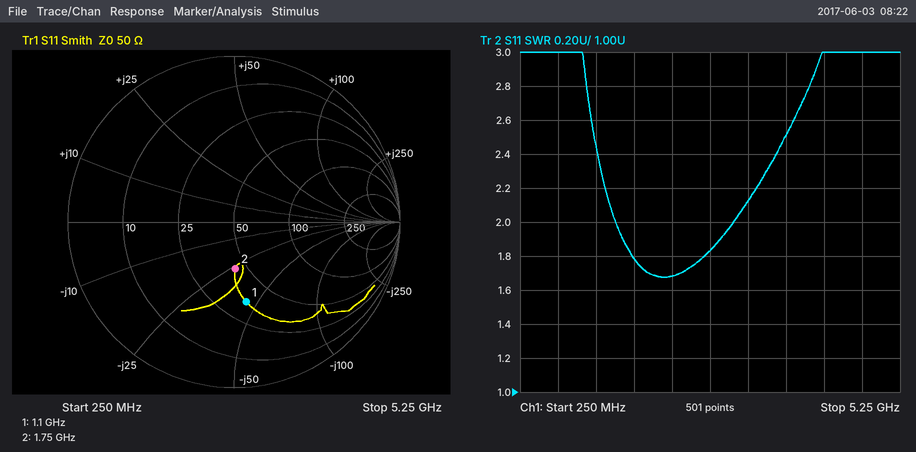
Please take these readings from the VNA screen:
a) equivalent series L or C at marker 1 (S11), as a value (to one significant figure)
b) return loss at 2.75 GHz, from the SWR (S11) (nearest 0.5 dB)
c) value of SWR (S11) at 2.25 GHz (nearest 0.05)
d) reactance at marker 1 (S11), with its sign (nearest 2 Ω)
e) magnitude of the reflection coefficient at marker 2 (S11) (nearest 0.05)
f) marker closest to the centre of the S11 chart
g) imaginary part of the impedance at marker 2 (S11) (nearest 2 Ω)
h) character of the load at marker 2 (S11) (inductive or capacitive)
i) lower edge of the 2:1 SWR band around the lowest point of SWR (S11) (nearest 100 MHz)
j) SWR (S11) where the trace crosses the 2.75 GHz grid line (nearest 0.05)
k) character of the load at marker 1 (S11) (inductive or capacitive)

3 pF
10.5 dB
1.70
-44 Ω
0.30
marker 2
-26 Ω
capacitive
1.5 GHz
1.85
capacitive
